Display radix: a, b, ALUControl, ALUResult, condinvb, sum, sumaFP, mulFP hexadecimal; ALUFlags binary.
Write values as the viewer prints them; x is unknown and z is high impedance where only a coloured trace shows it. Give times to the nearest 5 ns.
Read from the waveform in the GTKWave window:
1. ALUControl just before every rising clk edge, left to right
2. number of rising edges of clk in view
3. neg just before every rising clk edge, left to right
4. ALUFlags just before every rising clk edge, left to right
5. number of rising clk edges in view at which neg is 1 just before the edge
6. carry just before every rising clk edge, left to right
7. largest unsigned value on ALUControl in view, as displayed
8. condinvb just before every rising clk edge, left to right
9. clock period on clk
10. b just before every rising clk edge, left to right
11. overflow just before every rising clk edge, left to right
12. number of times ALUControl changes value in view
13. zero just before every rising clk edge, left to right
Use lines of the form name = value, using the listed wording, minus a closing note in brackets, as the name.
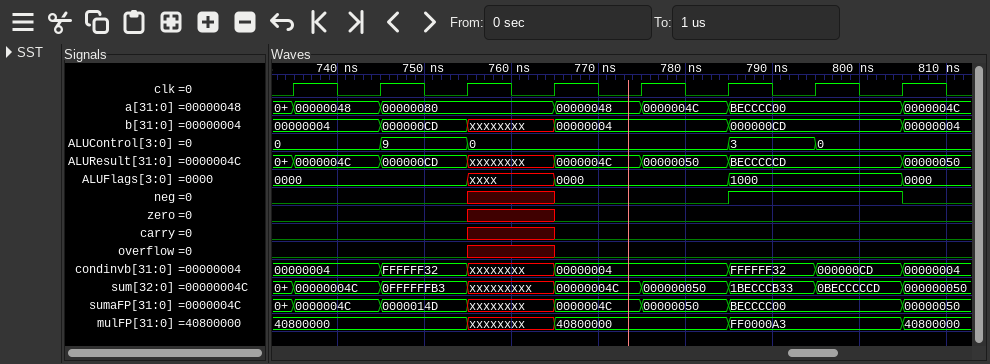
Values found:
ALUControl just before every rising clk edge, left to right = 0, 0, 9, 0, 0, 0, 3, 0
number of rising edges of clk in view = 8
neg just before every rising clk edge, left to right = 0 0 0 x 0 0 1 1
ALUFlags just before every rising clk edge, left to right = 0000, 0000, 0000, xxxx, 0000, 0000, 1000, 1000
number of rising clk edges in view at which neg is 1 just before the edge = 2
carry just before every rising clk edge, left to right = 0 0 0 x 0 0 0 0
largest unsigned value on ALUControl in view, as displayed = 9
condinvb just before every rising clk edge, left to right = 00000004, 00000004, FFFFFF32, xxxxxxxx, 00000004, 00000004, FFFFFF32, 000000CD
clock period on clk = 10 ns
b just before every rising clk edge, left to right = 00000004, 00000004, 000000CD, xxxxxxxx, 00000004, 00000004, 000000CD, 000000CD
overflow just before every rising clk edge, left to right = 0 0 0 x 0 0 0 0
number of times ALUControl changes value in view = 4
zero just before every rising clk edge, left to right = 0 0 0 x 0 0 0 0
